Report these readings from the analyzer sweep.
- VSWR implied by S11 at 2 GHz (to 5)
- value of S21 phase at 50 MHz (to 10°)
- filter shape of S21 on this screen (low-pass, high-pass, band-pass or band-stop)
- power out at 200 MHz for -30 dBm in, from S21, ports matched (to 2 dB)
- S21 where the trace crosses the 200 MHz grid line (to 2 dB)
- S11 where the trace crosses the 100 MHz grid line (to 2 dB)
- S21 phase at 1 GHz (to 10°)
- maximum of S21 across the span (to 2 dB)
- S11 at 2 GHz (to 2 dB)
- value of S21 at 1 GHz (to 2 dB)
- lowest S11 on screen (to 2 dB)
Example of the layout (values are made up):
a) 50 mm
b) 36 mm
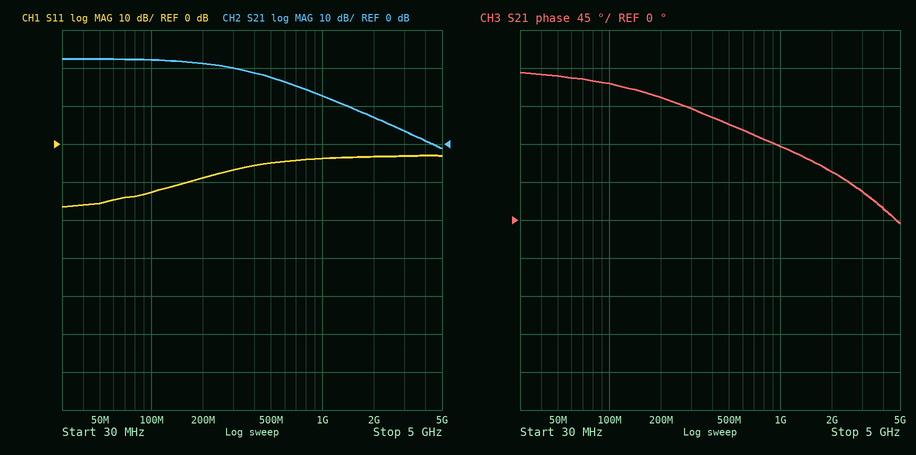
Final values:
a) 5
b) 170°
c) low-pass
d) -8 dBm
e) 22 dB
f) -12 dB
g) 90°
h) 22 dB
i) -4 dB
j) 12 dB
k) -16 dB
